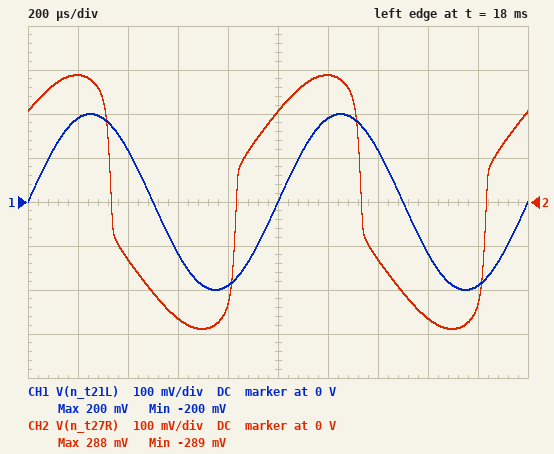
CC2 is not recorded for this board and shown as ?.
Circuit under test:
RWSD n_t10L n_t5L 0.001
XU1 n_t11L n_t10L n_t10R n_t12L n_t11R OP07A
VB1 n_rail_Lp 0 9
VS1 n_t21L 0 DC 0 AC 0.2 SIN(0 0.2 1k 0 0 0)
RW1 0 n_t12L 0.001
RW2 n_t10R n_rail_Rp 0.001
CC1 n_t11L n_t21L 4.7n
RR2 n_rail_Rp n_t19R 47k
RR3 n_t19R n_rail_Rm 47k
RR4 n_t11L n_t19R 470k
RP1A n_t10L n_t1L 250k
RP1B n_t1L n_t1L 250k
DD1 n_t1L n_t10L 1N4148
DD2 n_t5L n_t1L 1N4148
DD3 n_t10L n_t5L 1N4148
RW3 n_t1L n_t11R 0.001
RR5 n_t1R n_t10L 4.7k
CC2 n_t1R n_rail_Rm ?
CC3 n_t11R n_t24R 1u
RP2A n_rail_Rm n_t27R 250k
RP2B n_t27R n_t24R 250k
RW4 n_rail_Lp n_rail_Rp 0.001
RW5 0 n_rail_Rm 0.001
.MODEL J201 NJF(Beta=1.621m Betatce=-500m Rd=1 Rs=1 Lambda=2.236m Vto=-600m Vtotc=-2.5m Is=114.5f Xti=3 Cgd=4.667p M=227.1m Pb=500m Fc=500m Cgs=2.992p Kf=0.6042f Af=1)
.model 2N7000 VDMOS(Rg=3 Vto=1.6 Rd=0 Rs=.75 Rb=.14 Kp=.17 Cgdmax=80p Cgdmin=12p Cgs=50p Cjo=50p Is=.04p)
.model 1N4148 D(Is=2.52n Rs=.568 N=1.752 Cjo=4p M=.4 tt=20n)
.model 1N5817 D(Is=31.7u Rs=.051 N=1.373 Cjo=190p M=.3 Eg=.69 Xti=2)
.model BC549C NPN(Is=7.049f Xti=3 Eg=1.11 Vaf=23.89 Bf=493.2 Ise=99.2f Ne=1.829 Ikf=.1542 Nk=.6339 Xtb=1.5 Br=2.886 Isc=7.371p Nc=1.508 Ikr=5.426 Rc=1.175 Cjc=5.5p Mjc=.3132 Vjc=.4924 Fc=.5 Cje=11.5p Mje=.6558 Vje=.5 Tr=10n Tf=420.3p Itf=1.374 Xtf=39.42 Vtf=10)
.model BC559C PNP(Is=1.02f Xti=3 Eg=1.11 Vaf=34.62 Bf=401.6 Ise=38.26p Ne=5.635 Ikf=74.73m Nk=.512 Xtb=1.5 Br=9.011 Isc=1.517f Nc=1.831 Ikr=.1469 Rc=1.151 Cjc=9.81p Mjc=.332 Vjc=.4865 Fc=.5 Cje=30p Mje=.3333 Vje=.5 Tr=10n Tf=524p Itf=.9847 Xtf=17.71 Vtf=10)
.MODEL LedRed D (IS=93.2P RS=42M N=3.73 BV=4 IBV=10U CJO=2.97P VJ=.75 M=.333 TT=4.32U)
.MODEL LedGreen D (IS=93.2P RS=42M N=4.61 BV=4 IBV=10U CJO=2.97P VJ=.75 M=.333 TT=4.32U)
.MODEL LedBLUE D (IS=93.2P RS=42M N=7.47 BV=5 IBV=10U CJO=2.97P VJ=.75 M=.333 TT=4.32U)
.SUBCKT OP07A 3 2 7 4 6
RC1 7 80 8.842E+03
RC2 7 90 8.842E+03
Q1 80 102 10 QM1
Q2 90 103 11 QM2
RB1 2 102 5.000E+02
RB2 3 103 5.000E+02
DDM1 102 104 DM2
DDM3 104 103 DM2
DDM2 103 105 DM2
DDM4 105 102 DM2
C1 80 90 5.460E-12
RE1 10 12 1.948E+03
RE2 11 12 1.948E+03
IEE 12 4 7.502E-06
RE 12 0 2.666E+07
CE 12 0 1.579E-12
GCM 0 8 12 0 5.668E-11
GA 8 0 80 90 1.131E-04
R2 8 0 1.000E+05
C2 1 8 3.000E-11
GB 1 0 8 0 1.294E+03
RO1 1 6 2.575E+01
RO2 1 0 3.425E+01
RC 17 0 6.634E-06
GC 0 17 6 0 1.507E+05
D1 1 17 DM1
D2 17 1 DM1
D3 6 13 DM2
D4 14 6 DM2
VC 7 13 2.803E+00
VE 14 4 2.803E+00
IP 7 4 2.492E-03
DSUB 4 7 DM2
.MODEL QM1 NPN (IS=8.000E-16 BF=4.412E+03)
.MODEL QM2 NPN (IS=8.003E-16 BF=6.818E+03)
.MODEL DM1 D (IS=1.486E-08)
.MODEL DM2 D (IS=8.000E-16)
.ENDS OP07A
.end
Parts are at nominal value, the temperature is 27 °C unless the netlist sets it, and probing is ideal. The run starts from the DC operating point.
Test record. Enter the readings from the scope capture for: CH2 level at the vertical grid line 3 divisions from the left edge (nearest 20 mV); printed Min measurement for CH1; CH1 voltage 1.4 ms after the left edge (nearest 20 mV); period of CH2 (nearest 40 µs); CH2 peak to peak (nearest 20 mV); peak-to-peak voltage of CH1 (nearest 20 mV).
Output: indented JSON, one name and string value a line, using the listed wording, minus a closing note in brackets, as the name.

{
  "CH2 level at the vertical grid line 3 divisions from the left edge": "-260 mV",
  "printed Min measurement for CH1": "-200 mV",
  "CH1 voltage 1.4 ms after the left edge": "120 mV",
  "period of CH2": "1.00 ms",
  "CH2 peak to peak": "580 mV",
  "peak-to-peak voltage of CH1": "400 mV"
}
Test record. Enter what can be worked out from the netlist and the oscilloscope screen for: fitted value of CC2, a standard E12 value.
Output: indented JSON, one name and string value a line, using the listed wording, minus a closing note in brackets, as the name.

{
  "fitted value of CC2, a standard E12 value": "18 nF"
}
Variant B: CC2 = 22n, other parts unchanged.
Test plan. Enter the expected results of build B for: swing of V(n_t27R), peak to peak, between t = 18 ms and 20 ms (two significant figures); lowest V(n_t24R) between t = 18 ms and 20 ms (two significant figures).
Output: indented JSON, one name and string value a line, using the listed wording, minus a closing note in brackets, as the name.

{
  "swing of V(n_t27R), peak to peak, between t = 18 ms and 20 ms": "590 mV",
  "lowest V(n_t24R) between t = 18 ms and 20 ms": "-590 mV"
}
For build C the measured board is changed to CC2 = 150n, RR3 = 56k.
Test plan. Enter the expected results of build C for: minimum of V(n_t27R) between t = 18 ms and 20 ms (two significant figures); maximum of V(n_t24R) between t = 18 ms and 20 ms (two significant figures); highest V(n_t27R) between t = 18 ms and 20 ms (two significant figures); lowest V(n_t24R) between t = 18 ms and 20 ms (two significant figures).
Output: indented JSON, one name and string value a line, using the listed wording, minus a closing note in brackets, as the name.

{
  "minimum of V(n_t27R) between t = 18 ms and 20 ms": "-320 mV",
  "maximum of V(n_t24R) between t = 18 ms and 20 ms": "640 mV",
  "highest V(n_t27R) between t = 18 ms and 20 ms": "320 mV",
  "lowest V(n_t24R) between t = 18 ms and 20 ms": "-640 mV"
}
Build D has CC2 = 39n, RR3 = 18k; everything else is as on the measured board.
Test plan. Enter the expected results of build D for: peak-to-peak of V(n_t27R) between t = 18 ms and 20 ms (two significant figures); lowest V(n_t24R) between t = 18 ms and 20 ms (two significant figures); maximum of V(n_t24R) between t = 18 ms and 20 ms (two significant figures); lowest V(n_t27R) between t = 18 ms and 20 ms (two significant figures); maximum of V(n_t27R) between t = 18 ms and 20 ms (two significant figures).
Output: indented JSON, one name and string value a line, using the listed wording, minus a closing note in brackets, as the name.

{
  "peak-to-peak of V(n_t27R) between t = 18 ms and 20 ms": "550 mV",
  "lowest V(n_t24R) between t = 18 ms and 20 ms": "-490 mV",
  "maximum of V(n_t24R) between t = 18 ms and 20 ms": "610 mV",
  "lowest V(n_t27R) between t = 18 ms and 20 ms": "-250 mV",
  "maximum of V(n_t27R) between t = 18 ms and 20 ms": "310 mV"
}
